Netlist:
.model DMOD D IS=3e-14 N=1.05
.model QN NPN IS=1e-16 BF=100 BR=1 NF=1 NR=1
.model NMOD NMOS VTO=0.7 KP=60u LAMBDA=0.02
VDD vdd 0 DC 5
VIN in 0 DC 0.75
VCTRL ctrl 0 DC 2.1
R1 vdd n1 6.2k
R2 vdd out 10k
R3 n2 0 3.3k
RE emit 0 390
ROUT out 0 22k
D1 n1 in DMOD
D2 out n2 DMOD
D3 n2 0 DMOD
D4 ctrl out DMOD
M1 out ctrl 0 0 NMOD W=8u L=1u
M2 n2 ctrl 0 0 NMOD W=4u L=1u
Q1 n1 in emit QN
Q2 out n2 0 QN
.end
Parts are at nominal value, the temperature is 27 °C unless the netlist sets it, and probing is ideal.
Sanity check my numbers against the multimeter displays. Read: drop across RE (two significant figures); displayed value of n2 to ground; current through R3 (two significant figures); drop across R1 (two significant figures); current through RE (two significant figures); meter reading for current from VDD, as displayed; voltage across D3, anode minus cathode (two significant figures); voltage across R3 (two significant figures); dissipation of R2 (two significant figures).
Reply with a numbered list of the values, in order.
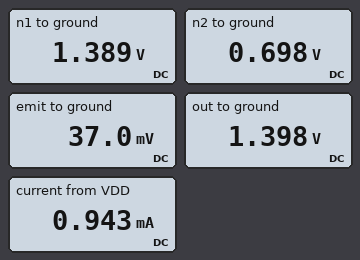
1. 37 mV
2. 0.698 V
3. 210 µA
4. 3.6 V
5. 95 µA
6. 0.943 mA
7. 700 mV
8. 700 mV
9. 1.3 mW
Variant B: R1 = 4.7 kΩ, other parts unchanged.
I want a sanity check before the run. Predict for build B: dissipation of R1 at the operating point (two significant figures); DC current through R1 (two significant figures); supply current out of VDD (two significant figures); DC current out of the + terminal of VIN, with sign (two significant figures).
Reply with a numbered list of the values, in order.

1. 2.8 mW
2. 770 µA
3. 1.1 mA
4. -670 µA
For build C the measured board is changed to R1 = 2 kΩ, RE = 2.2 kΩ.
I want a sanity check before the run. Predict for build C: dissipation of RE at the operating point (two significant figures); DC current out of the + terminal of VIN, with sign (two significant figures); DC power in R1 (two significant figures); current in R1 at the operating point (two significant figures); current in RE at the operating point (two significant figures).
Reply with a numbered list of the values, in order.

1. 2.0 µW
2. -1.8 mA
3. 6.4 mW
4. 1.8 mA
5. 30 µA
